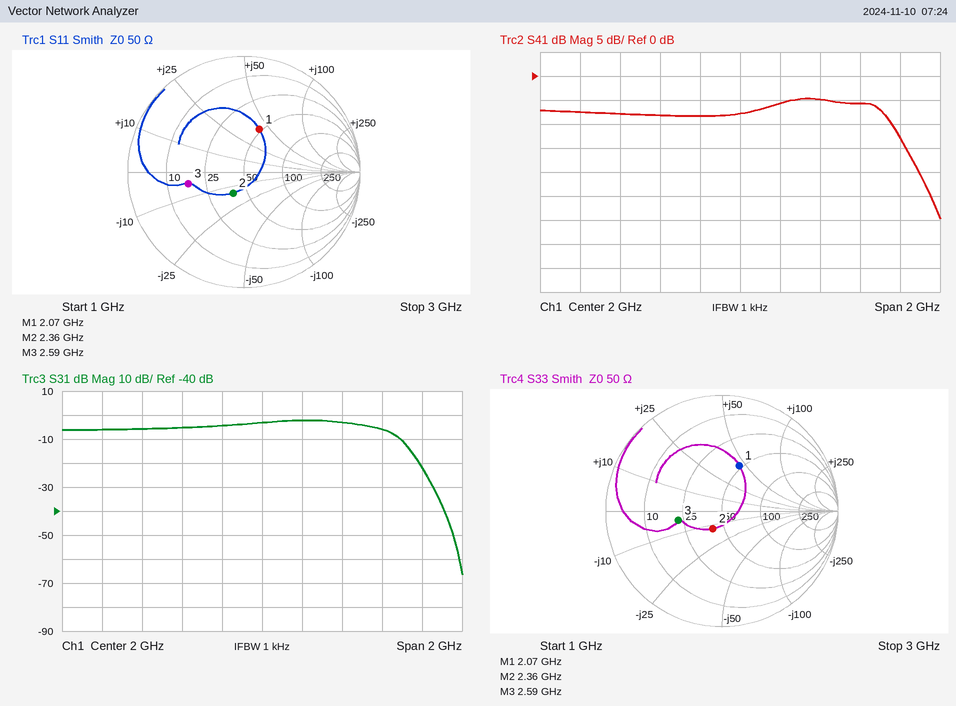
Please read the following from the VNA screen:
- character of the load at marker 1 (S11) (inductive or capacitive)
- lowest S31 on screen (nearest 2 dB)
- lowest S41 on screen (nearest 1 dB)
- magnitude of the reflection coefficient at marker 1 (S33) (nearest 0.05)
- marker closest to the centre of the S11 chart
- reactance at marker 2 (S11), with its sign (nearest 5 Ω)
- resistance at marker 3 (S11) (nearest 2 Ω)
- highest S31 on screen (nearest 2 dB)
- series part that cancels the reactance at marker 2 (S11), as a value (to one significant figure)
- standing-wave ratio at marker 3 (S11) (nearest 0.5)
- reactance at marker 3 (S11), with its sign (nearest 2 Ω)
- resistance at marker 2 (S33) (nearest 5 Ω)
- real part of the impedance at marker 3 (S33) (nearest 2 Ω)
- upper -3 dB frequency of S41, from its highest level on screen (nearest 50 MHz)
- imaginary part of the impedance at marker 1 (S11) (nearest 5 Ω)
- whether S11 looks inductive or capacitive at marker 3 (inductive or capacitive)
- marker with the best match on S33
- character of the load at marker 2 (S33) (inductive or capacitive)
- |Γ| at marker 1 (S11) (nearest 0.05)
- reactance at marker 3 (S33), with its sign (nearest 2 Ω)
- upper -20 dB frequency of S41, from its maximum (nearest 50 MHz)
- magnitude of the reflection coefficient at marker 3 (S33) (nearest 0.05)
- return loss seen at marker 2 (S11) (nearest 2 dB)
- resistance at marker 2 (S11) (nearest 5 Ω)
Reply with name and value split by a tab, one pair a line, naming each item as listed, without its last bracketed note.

character of the load at marker 1 (S11)	inductive
lowest S31 on screen	-66 dB
lowest S41 on screen	-30 dB
magnitude of the reflection coefficient at marker 1 (S33)	0.40
marker closest to the centre of the S11 chart	marker 2
reactance at marker 2 (S11), with its sign	-15 Ω
resistance at marker 3 (S11)	18 Ω
highest S31 on screen	-2 dB
series part that cancels the reactance at marker 2 (S11), as a value	1 nH
standing-wave ratio at marker 3 (S11)	3.0
reactance at marker 3 (S11), with its sign	-4 Ω
resistance at marker 2 (S33)	40 Ω
real part of the impedance at marker 3 (S33)	22 Ω
upper -3 dB frequency of S41, from its highest level on screen	2.70 GHz
imaginary part of the impedance at marker 1 (S11)	+40 Ω
whether S11 looks inductive or capacitive at marker 3	capacitive
marker with the best match on S33	marker 2
character of the load at marker 2 (S33)	capacitive
|Γ| at marker 1 (S11)	0.40
reactance at marker 3 (S33), with its sign	-4 Ω
upper -20 dB frequency of S41, from its maximum	2.95 GHz
magnitude of the reflection coefficient at marker 3 (S33)	0.40
return loss seen at marker 2 (S11)	14 dB
resistance at marker 2 (S11)	40 Ω
